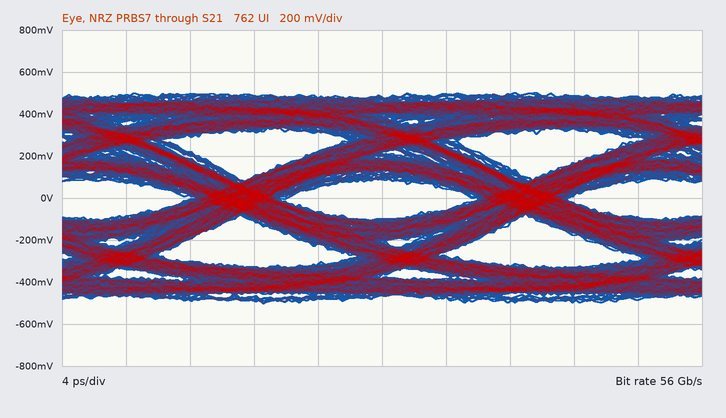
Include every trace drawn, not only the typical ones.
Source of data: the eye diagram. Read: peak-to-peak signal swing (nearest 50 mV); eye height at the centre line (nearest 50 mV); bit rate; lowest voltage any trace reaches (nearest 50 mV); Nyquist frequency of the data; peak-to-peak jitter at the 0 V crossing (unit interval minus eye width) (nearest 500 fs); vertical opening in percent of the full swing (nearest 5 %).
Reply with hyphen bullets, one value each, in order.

- 1.00 V
- 200 mV
- 56 Gb/s
- -500 mV
- 28 GHz
- 6.5 ps
- 20 %
